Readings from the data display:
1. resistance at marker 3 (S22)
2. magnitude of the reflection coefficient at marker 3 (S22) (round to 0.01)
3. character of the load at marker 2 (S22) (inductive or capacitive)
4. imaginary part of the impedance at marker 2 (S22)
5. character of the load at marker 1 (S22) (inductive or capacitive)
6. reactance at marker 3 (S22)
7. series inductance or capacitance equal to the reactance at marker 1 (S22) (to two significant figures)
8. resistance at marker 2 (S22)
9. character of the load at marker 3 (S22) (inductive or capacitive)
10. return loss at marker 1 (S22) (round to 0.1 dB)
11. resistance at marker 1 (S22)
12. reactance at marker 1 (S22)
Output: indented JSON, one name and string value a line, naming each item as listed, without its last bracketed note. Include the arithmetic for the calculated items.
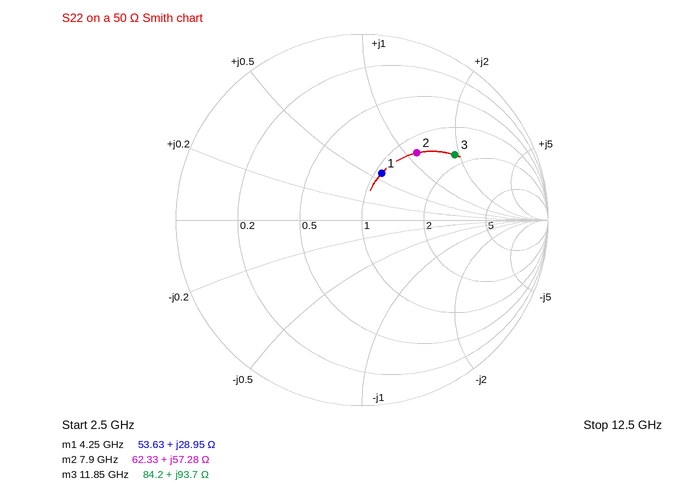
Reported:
{
  "resistance at marker 3": "84.2 Ω",
  "magnitude of the reflection coefficient at marker 3 (S22)": "0.61",
  "character of the load at marker 2 (S22)": "inductive",
  "imaginary part of the impedance at marker 2": "+57.28 Ω",
  "character of the load at marker 1 (S22)": "inductive",
  "reactance at marker 3": "+93.7 Ω",
  "series inductance or capacitance equal to the reactance at marker 1 (S22)": "L = 28.95 Ω/(2π × 4.25 GHz) ≈ 1.1 nH",
  "resistance at marker 2": "62.33 Ω",
  "character of the load at marker 3 (S22)": "inductive",
  "return loss at marker 1 (S22)": "11.3 dB",
  "resistance at marker 1": "53.63 Ω",
  "reactance at marker 1": "+28.95 Ω"
}
